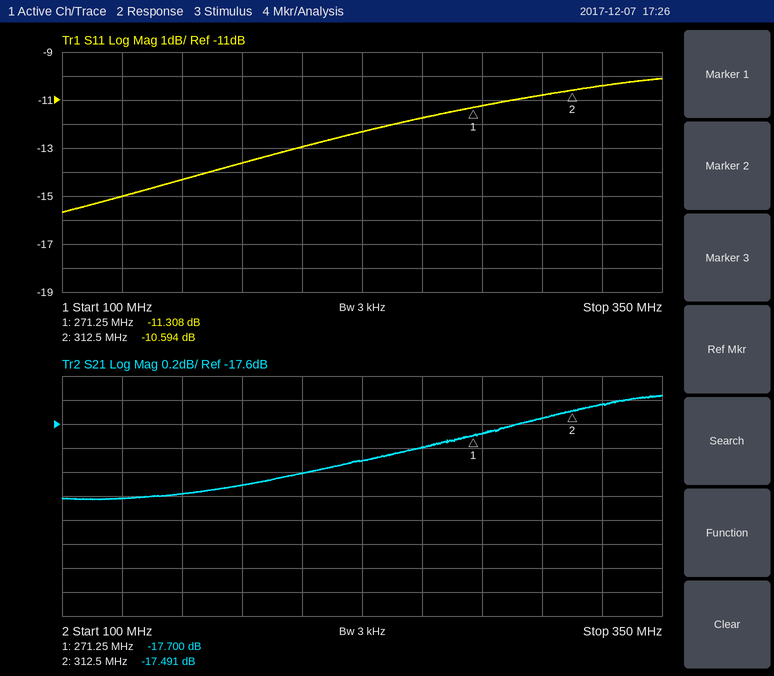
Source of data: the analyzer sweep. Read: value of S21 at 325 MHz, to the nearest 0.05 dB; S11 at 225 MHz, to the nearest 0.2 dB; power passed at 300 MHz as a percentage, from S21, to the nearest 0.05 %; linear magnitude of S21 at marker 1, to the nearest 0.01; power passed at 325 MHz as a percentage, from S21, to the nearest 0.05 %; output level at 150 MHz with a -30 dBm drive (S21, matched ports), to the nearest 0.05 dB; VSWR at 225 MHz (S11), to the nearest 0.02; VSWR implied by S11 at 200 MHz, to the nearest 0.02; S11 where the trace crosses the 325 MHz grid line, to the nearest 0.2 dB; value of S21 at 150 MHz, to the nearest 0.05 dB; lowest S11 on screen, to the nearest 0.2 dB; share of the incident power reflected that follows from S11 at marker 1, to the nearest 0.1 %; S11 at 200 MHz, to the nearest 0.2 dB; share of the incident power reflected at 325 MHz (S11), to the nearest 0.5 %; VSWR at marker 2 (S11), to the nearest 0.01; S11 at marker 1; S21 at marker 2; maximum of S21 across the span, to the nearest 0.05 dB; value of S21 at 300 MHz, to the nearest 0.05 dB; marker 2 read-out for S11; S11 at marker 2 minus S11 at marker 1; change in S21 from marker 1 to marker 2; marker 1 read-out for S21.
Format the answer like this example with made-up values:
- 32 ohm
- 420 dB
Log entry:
- -17.45 dB
- -12.4 dB
- 1.75 %
- 0.13
- 1.80 %
- -48.20 dBm
- 1.64
- 1.58
- -10.4 dB
- -18.20 dB
- -15.6 dB
- 7.4 %
- -13.0 dB
- 9.0 %
- 1.84
- -11.308 dB
- -17.491 dB
- -17.35 dB
- -17.55 dB
- -10.594 dB
- 0.714 dB
- 0.209 dB
- -17.700 dB
